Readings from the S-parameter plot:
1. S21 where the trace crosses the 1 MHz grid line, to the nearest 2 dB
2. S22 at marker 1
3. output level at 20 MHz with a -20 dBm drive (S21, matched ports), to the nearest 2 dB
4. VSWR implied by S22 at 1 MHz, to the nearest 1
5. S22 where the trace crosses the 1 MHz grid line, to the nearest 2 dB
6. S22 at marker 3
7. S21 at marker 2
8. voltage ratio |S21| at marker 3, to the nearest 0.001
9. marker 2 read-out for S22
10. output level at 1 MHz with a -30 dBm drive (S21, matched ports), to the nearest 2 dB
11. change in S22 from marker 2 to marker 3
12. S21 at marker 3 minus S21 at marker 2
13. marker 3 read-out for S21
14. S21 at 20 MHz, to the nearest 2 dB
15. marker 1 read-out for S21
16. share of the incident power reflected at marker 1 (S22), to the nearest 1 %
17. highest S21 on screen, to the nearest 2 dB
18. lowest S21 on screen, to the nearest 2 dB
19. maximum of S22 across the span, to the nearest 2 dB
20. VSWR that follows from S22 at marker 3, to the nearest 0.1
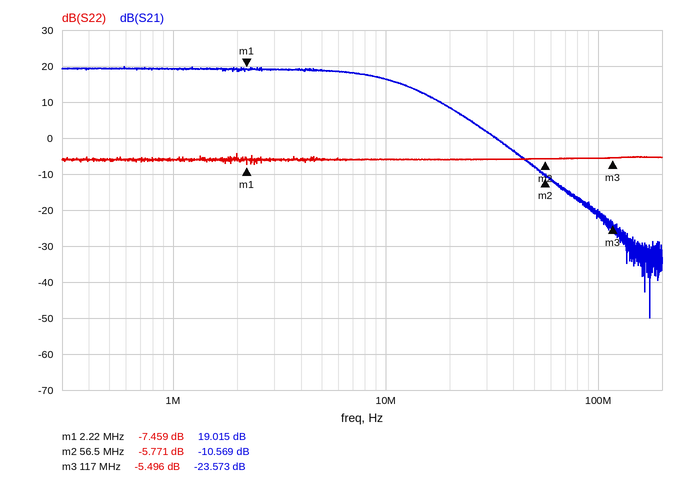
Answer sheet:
20 dB
-7.459 dB
-12 dBm
3
-6 dB
-5.496 dB
-10.569 dB
0.066
-5.771 dB
-10 dBm
0.275 dB
-13.004 dB
-23.573 dB
8 dB
19.015 dB
18 %
20 dB
-50 dB
-4 dB
3.3
